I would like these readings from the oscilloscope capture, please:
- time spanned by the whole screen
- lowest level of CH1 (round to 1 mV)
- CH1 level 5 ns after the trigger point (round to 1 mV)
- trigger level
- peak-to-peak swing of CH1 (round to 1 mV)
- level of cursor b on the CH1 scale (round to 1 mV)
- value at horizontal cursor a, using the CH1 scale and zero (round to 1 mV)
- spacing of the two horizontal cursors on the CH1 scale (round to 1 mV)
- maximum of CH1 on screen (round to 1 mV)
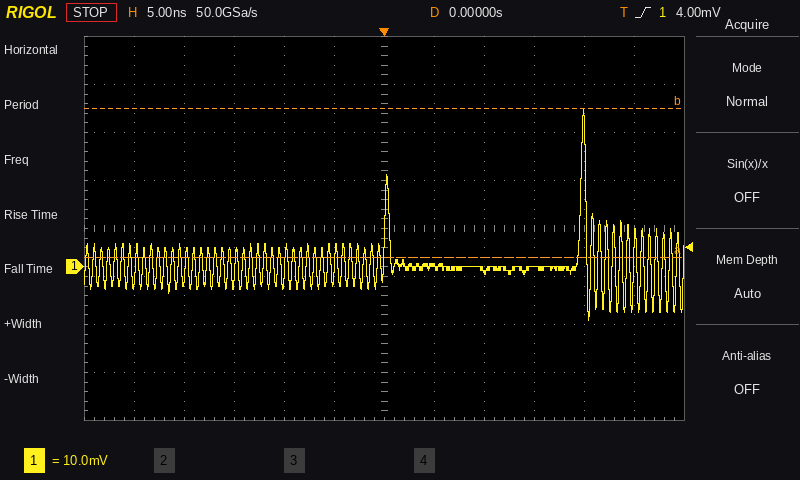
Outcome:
60 ns
-11 mV
0 mV
4.00 mV
44 mV
33 mV
2 mV
31 mV
33 mV
